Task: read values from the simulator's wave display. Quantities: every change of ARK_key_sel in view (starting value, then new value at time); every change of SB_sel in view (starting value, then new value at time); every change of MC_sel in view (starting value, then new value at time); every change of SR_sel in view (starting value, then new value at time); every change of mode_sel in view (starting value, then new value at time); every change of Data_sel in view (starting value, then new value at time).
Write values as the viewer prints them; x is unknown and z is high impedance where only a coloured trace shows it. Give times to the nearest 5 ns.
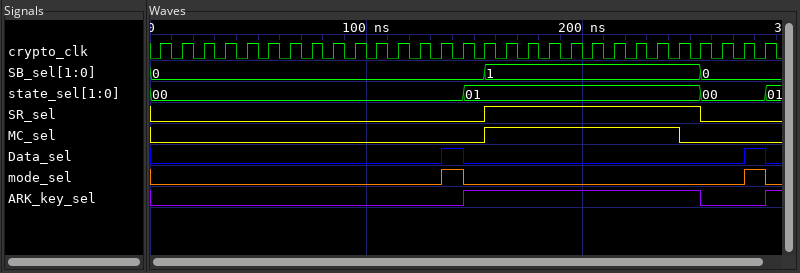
0, 1 at 145 ns, 0 at 255 ns, 1 at 285 ns
0, 1 at 155 ns, 0 at 255 ns
0, 1 at 155 ns, 0 at 245 ns
0, 1 at 155 ns, 0 at 255 ns
0, 1 at 135 ns, 0 at 145 ns, 1 at 275 ns, 0 at 285 ns
0, 1 at 135 ns, 0 at 145 ns, 1 at 275 ns, 0 at 285 ns
